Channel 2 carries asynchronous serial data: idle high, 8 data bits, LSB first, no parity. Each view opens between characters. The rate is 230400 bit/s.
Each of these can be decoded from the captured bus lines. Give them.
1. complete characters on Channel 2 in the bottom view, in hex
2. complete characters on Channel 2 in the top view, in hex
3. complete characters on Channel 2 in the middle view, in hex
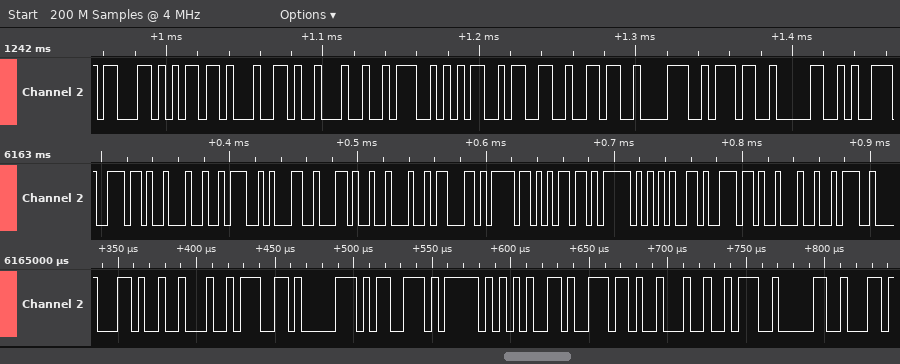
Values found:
2C, 22, 67, 70, 73, 5F, 65, 6E, 22, 3A, 30
63, 6D, 64, 22, 3A, 35, 33, 36, 38, 37, 30
6E, 22, 3A, 31, 2C, 22, 63, 6F, 6D, 5F, 65, 6E, 22, 3A
